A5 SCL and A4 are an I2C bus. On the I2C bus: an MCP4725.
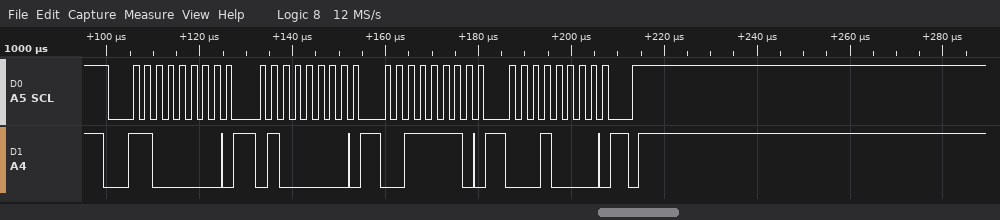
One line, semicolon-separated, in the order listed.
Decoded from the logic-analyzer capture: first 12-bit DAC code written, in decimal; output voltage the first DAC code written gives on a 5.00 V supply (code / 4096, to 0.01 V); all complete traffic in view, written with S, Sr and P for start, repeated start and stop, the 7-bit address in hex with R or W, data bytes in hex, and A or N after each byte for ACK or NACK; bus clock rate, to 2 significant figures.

993; 1.21 V; S 60W A 40 A 3E A 10 A P; 400 kHz
